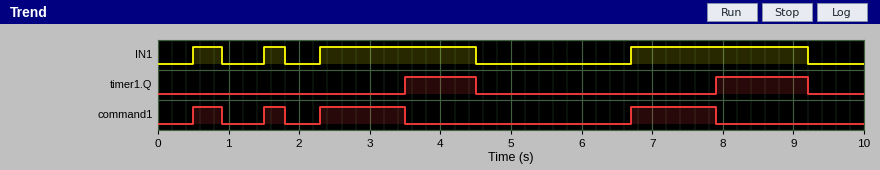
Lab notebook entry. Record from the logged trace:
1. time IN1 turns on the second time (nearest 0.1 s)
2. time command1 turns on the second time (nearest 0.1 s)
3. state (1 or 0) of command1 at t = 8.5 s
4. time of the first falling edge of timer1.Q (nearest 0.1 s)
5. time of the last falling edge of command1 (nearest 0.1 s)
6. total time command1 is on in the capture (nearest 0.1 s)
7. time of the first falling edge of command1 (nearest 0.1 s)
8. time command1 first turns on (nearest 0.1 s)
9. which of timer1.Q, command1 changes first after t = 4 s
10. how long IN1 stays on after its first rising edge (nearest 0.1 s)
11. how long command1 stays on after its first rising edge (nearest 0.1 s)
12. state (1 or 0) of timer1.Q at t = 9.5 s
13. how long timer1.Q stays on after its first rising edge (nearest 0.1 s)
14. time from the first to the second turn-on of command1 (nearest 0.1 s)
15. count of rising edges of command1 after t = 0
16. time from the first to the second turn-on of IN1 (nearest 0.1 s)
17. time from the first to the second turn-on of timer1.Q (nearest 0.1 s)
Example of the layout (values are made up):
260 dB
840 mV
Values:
1.5 s
1.5 s
0
4.5 s
7.9 s
3.1 s
0.9 s
0.5 s
timer1.Q
0.4 s
0.4 s
0
1.0 s
1.0 s
4
1.0 s
4.4 s
